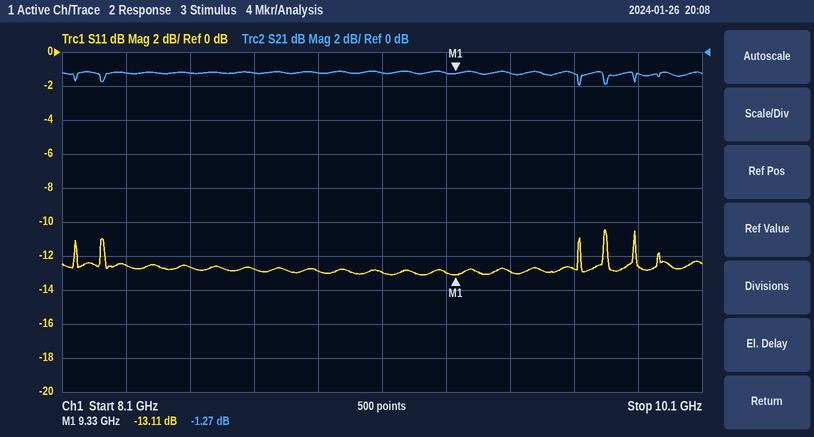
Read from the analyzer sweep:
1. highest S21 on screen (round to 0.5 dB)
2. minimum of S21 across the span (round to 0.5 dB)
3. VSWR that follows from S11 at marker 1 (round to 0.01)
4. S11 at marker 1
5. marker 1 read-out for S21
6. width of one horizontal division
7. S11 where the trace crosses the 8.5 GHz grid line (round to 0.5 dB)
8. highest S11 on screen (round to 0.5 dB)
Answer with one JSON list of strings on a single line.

["-1.0 dB", "-2.0 dB", "1.57", "-13.11 dB", "-1.27 dB", "200 MHz", "-12.5 dB", "-10.5 dB"]
